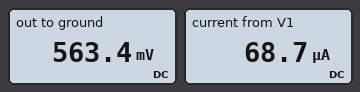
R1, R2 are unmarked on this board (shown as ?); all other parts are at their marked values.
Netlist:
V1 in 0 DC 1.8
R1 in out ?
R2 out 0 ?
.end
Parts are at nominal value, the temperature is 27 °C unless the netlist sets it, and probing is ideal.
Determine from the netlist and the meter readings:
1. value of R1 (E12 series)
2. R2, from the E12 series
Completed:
18 kΩ
8.2 kΩ
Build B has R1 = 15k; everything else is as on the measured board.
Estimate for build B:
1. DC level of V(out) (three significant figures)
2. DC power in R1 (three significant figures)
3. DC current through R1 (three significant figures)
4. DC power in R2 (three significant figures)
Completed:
636 mV
90.3 µW
77.6 µA
49.4 µW
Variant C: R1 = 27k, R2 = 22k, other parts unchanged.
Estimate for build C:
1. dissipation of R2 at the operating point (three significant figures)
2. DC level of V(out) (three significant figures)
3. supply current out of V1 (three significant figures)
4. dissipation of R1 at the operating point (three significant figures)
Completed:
29.7 µW
808 mV
36.7 µA
36.4 µW
